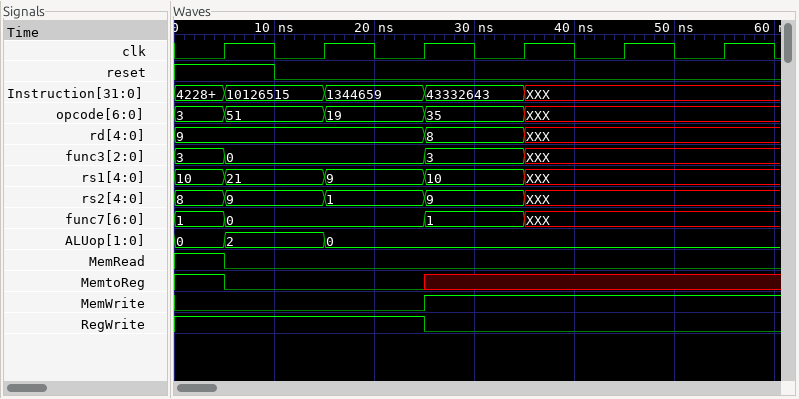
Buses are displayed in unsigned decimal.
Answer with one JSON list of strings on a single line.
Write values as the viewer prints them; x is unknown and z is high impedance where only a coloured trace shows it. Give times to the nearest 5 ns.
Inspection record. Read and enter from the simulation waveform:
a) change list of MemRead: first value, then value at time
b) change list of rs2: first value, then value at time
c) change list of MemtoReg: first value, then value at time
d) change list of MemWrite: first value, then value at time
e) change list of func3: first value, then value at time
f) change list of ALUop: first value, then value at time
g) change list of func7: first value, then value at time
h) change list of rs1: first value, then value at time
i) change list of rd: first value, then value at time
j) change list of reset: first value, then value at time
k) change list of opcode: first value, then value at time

["1, 0 at 5 ns", "8, 9 at 5 ns, 1 at 15 ns, 9 at 25 ns, XXX at 35 ns", "1, 0 at 5 ns, x at 25 ns", "0, 1 at 25 ns", "3, 0 at 5 ns, 3 at 25 ns, XXX at 35 ns", "0, 2 at 5 ns, 0 at 15 ns", "1, 0 at 5 ns, 1 at 25 ns, XXX at 35 ns", "10, 21 at 5 ns, 9 at 15 ns, 10 at 25 ns, XXX at 35 ns", "9, 8 at 25 ns, XXX at 35 ns", "1, 0 at 10 ns", "3, 51 at 5 ns, 19 at 15 ns, 35 at 25 ns, XXX at 35 ns"]
